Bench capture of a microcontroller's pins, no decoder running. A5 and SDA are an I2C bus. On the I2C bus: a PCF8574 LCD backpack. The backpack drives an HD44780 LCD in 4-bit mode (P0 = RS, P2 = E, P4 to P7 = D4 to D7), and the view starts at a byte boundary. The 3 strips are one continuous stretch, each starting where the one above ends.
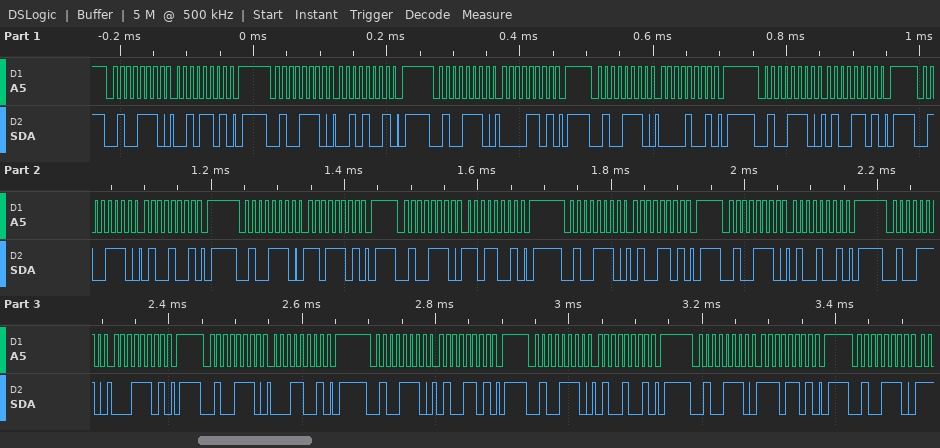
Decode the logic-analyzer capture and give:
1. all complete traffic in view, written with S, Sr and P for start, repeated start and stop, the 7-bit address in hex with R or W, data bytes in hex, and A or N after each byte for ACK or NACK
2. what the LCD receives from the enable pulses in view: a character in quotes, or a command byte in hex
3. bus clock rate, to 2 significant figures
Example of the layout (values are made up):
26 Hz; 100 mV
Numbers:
S 27W A 2D A P S 27W A 29 A P S 27W A 0D A P S 27W A 09 A P S 27W A 4D A P S 27W A 49 A P S 27W A DD A P S 27W A D9 A P S 27W A 4D A P S 27W A 49 A P S 27W A 1D A P S 27W A 19 A P S 27W A 4D A P S 27W A 49 A P S 27W A ED A P S 27W A; ' ' 'M' 'A'; 100 kHz
